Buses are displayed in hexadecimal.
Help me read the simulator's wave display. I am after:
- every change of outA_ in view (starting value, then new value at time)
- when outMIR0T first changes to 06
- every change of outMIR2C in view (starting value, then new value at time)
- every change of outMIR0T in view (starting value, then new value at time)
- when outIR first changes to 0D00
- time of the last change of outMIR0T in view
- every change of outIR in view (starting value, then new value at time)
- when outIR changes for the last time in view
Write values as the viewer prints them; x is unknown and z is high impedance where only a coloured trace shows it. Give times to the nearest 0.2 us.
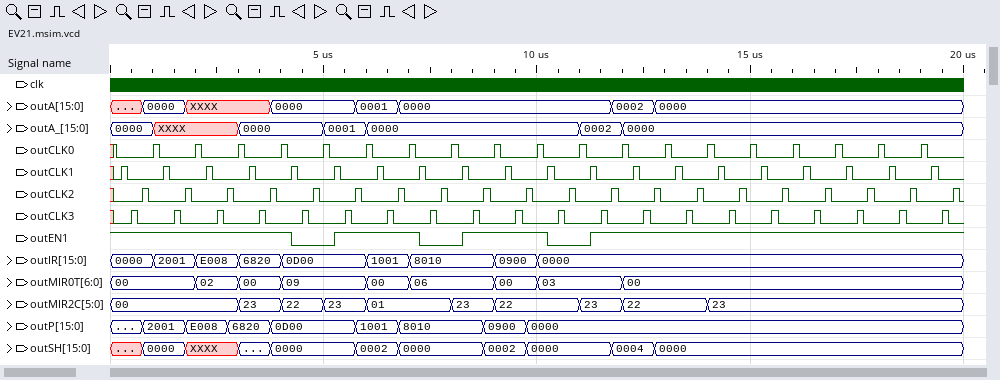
0000, XXXX at 1 us, 0000 at 3 us, 0001 at 5 us, 0000 at 6 us, 0002 at 11 us, 0000 at 12 us
7 us
00, 23 at 3 us, 22 at 4 us, 23 at 5 us, 01 at 6 us, 23 at 8 us, 22 at 9 us, 23 at 11 us, 22 at 12 us, 23 at 14 us
00, 02 at 2 us, 00 at 3 us, 09 at 4 us, 00 at 6 us, 06 at 7 us, 00 at 9 us, 03 at 10 us, 00 at 12 us
4 us
12 us
0000, 2001 at 1 us, E008 at 2 us, 6820 at 3 us, 0D00 at 4 us, 1001 at 6 us, 8010 at 7 us, 0900 at 9 us, 0000 at 10 us
10 us
